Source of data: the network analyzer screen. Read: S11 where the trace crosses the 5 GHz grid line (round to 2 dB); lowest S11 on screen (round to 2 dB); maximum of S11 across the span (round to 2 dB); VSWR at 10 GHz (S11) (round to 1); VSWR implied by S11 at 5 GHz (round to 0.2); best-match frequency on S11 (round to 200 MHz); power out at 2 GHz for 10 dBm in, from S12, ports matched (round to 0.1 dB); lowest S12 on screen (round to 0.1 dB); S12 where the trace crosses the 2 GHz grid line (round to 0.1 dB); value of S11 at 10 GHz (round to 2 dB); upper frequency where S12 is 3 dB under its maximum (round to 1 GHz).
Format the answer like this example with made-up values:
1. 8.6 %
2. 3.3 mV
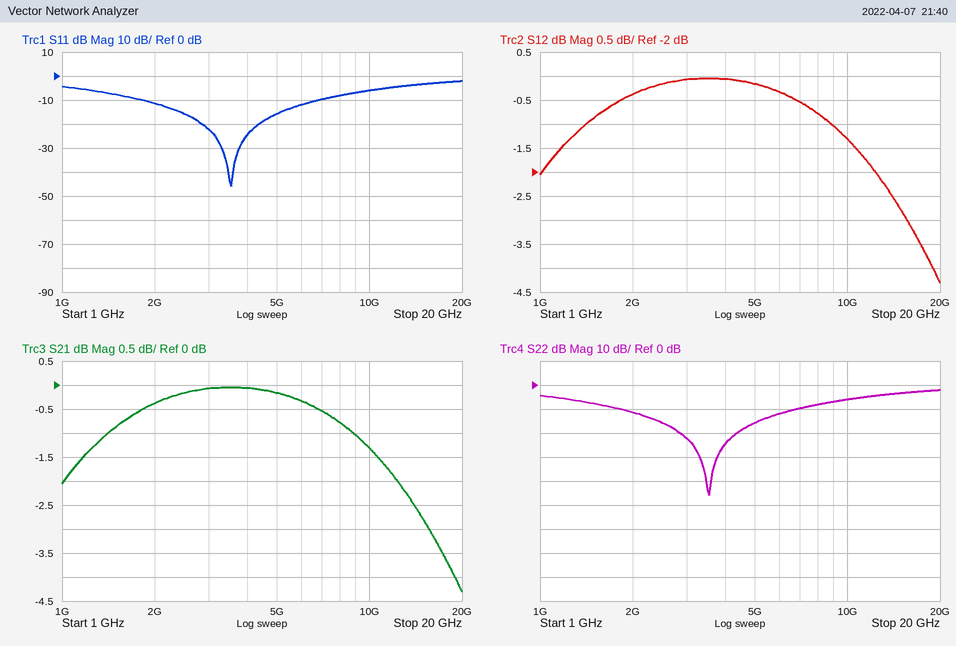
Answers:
1. -16 dB
2. -46 dB
3. -2 dB
4. 3
5. 1.4
6. 3.6 GHz
7. 9.6 dBm
8. -4.3 dB
9. -0.4 dB
10. -6 dB
11. 16 GHz
